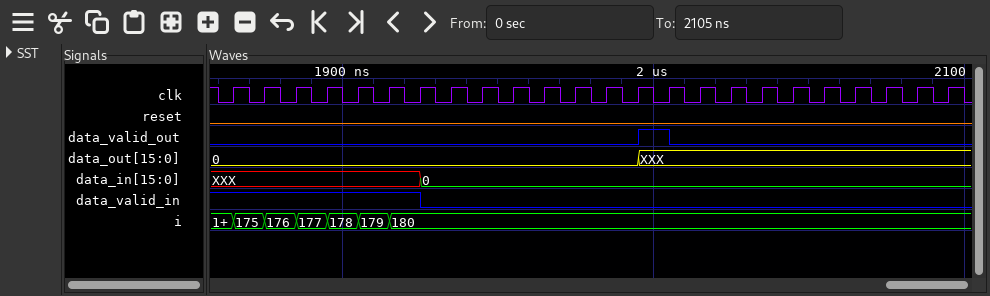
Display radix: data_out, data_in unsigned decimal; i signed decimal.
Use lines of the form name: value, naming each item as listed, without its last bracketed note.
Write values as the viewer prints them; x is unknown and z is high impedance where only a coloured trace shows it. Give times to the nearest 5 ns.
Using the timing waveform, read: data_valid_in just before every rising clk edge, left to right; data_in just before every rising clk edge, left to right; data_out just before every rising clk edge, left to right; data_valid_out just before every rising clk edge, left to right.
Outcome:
data_valid_in just before every rising clk edge, left to right: 1 1 1 1 1 1 1 0 0 0 0 0 0 0 0 0 0 0 0 0 0 0 0 0
data_in just before every rising clk edge, left to right: XXX, XXX, XXX, XXX, XXX, XXX, XXX, 0, 0, 0, 0, 0, 0, 0, 0, 0, 0, 0, 0, 0, 0, 0, 0, 0
data_out just before every rising clk edge, left to right: 0, 0, 0, 0, 0, 0, 0, 0, 0, 0, 0, 0, 0, 0, XXX, XXX, XXX, XXX, XXX, XXX, XXX, XXX, XXX, XXX
data_valid_out just before every rising clk edge, left to right: 0 0 0 0 0 0 0 0 0 0 0 0 0 0 1 0 0 0 0 0 0 0 0 0
